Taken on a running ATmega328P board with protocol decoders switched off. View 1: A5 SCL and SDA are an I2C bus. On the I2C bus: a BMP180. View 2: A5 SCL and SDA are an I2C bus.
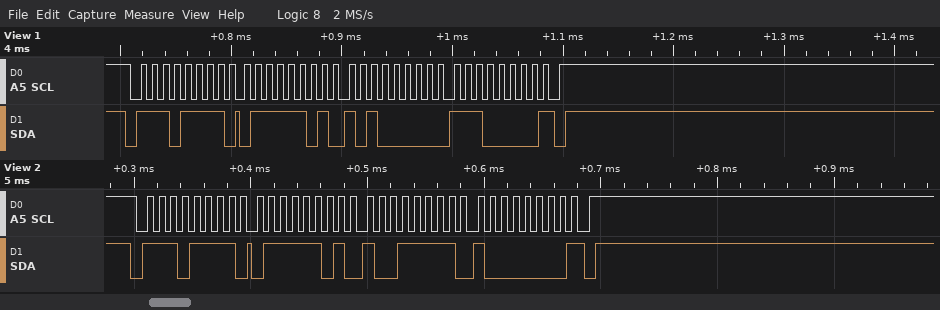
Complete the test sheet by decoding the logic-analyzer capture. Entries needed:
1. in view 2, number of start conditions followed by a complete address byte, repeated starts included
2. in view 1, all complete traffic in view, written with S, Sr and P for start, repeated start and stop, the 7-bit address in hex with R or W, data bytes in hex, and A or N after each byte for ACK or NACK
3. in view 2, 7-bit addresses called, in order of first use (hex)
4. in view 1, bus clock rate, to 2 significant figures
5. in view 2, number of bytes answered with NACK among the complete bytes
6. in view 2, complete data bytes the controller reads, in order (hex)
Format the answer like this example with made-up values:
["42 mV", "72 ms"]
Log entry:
["1", "S 77R A 7D A A0 A E0 N P", "0x77", "100 kHz", "1", "7D 9F 80"]
